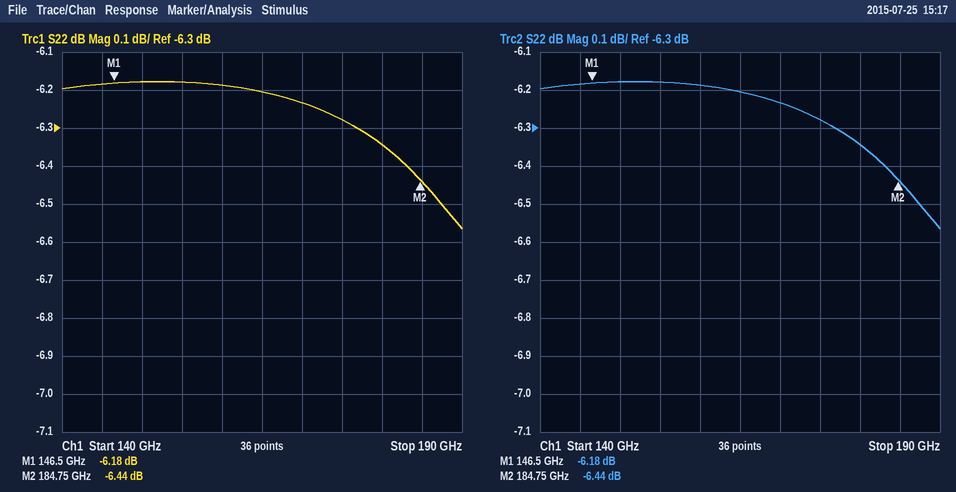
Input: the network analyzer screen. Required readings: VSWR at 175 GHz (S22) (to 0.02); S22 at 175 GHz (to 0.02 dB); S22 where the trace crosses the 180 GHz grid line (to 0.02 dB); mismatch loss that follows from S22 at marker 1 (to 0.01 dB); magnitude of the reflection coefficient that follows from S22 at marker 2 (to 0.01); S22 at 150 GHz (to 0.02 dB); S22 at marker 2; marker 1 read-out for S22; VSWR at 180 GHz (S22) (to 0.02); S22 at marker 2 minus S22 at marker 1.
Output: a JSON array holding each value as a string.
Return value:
["2.88", "-6.28 dB", "-6.34 dB", "1.20 dB", "0.48", "-6.18 dB", "-6.44 dB", "-6.18 dB", "2.86", "-0.26 dB"]
